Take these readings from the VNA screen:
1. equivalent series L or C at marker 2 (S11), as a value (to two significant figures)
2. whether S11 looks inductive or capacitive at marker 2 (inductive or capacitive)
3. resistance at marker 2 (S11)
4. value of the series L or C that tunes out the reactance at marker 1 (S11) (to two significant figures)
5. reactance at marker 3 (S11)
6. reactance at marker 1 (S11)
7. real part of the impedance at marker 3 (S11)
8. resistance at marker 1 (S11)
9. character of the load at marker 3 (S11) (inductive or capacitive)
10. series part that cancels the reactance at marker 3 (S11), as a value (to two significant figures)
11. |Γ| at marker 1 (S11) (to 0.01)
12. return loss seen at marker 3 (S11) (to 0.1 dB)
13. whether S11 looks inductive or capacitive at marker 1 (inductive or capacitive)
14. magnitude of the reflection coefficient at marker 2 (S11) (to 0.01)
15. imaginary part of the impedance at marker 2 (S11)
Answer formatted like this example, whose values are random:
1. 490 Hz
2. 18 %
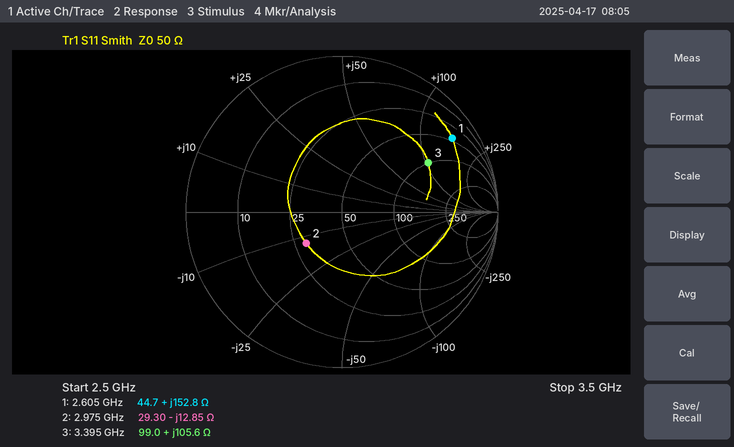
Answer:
1. 4.2 pF
2. capacitive
3. 29.30 Ω
4. 400 fF
5. +105.6 Ω
6. +152.8 Ω
7. 99.0 Ω
8. 44.7 Ω
9. inductive
10. 440 fF
11. 0.85
12. 3.9 dB
13. inductive
14. 0.30
15. -12.85 Ω
